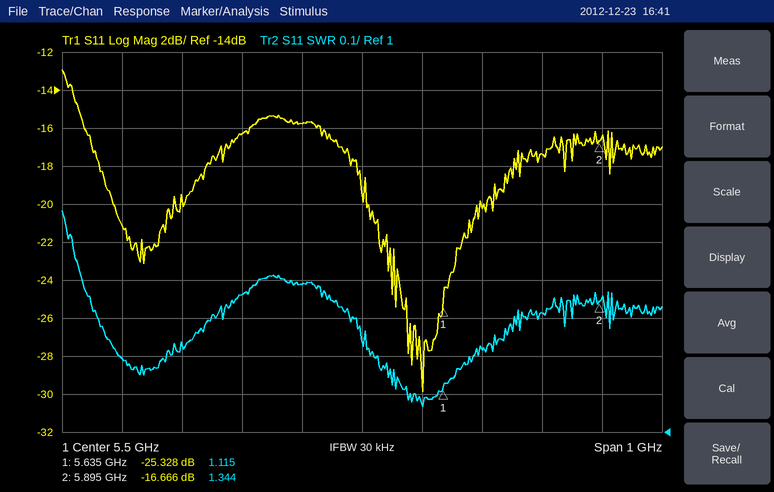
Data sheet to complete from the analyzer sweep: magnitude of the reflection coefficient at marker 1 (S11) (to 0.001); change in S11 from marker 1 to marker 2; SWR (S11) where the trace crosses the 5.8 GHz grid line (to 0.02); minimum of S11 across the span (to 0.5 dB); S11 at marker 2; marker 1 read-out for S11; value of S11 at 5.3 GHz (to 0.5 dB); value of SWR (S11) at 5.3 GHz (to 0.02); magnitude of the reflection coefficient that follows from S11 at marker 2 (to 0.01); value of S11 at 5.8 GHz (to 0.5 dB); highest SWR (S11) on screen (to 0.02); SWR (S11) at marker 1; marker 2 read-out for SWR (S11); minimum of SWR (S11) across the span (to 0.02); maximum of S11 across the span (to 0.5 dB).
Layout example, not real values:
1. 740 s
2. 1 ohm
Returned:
1. 0.054
2. 8.662 dB
3. 1.32
4. -30.0 dB
5. -16.666 dB
6. -25.328 dB
7. -16.5 dB
8. 1.36
9. 0.15
10. -17.5 dB
11. 1.58
12. 1.115
13. 1.344
14. 1.06
15. -13.0 dB
